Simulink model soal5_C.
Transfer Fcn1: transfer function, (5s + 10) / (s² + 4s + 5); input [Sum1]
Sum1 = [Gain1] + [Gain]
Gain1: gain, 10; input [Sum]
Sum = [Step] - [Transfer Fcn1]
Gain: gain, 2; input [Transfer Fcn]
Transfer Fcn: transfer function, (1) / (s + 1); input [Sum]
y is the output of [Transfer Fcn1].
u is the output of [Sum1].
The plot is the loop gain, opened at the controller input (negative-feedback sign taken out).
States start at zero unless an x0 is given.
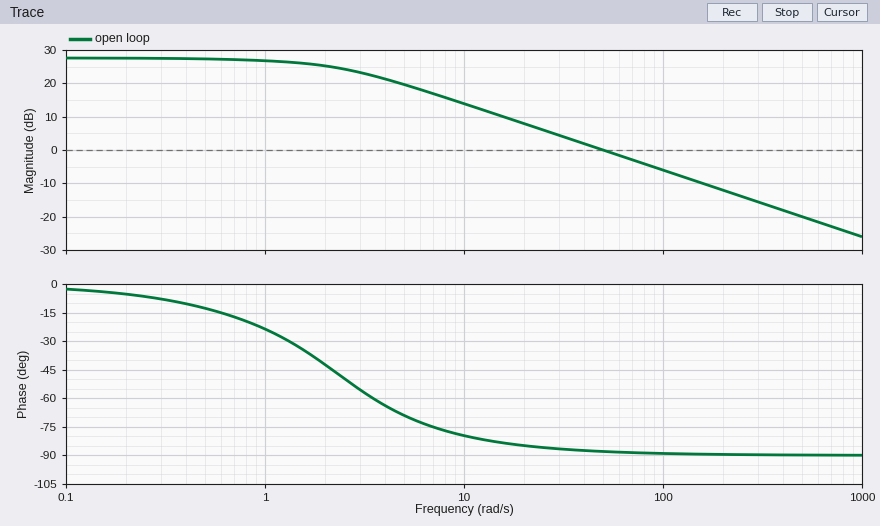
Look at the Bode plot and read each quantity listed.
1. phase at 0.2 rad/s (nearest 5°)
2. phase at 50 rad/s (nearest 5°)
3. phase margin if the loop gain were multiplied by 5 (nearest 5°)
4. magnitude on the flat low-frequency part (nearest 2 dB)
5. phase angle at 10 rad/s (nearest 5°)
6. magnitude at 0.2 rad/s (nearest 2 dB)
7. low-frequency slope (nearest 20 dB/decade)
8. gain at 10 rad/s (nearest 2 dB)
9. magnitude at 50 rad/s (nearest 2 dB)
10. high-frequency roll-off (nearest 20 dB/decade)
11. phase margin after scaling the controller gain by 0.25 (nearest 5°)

-5°
-90°
90°
28 dB
-80°
28 dB
0 dB/decade
14 dB
0 dB
-20 dB/decade
100°
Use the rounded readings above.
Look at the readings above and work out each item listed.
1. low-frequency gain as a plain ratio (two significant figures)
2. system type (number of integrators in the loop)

25
0
